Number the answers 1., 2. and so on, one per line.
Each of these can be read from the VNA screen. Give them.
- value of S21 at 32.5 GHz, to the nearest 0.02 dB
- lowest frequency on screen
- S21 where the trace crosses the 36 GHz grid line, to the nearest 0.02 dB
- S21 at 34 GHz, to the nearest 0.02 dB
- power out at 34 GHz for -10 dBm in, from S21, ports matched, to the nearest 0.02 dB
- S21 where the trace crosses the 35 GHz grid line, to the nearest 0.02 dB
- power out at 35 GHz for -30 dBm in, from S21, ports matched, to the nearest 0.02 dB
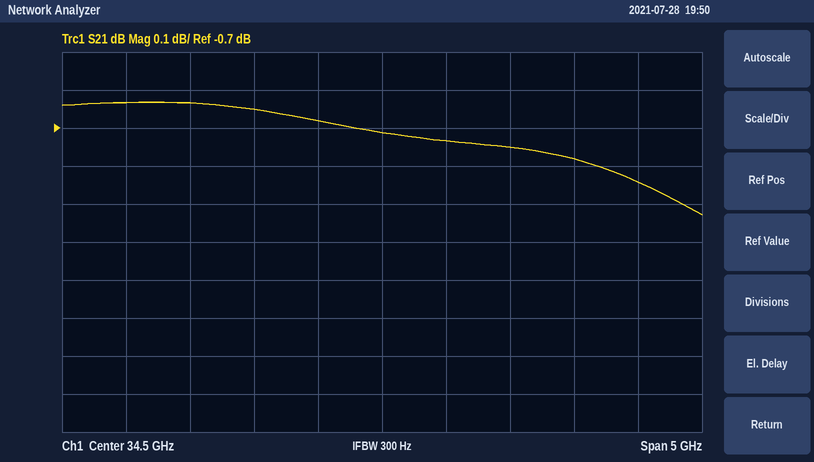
1. -0.64 dB
2. 32 GHz
3. -0.78 dB
4. -0.68 dB
5. -10.68 dBm
6. -0.74 dB
7. -30.74 dBm
